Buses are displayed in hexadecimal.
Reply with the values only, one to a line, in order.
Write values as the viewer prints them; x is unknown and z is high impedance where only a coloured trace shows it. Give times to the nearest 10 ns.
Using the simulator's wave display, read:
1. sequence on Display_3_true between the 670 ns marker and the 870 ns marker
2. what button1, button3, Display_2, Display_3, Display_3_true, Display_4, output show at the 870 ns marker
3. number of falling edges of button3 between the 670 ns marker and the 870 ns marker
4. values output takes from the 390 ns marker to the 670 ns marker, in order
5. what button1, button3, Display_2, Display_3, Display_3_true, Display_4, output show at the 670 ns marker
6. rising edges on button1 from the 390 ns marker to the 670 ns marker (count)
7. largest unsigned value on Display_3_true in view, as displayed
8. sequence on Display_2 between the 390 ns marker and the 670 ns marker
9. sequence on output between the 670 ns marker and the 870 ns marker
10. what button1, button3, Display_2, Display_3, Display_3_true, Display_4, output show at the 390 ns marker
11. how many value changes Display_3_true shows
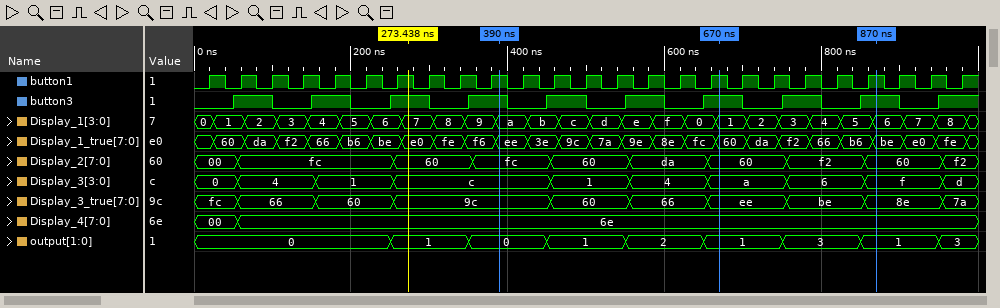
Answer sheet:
ee, be, 8e
button1=1, button3=1, Display_2=60, Display_3=f, Display_3_true=8e, Display_4=6e, output=1
2
0, 1, 2, 1
button1=1, button3=1, Display_2=60, Display_3=a, Display_3_true=ee, Display_4=6e, output=1
7
fc
fc, 60, da, 60
1, 3, 1
button1=1, button3=1, Display_2=fc, Display_3=c, Display_3_true=9c, Display_4=6e, output=0
9
